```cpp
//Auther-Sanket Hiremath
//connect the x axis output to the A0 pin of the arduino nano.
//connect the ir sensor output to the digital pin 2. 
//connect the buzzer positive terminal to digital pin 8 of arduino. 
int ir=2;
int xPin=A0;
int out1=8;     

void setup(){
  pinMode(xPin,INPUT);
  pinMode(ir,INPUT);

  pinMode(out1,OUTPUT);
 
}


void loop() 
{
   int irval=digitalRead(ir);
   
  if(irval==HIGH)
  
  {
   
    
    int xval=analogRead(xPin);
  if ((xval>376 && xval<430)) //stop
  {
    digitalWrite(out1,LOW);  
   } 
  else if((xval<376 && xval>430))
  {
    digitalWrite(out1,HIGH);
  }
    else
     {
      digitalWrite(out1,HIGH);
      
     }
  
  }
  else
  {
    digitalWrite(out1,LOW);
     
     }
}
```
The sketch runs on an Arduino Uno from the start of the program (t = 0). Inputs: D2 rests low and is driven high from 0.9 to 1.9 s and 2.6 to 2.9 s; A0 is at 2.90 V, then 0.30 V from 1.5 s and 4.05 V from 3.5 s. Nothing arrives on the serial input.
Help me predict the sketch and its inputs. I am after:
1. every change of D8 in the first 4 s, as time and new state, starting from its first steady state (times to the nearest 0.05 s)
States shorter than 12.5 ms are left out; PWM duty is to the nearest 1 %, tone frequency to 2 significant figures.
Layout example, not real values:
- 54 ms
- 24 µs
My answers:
- 0 s low; 0.9 s high; 1.9 s low; 2.6 s high; 2.9 s low
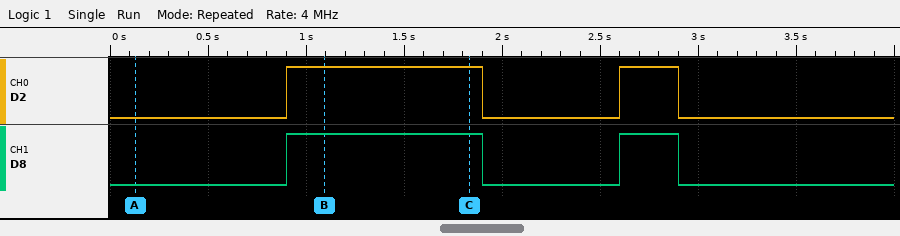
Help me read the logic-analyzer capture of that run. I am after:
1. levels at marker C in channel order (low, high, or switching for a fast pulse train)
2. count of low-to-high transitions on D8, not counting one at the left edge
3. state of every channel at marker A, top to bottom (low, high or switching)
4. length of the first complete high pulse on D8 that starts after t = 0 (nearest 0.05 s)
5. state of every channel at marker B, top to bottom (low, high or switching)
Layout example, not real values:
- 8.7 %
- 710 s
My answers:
- D2 high, D8 high
- 2
- D2 low, D8 low
- 1.00 s
- D2 high, D8 high
